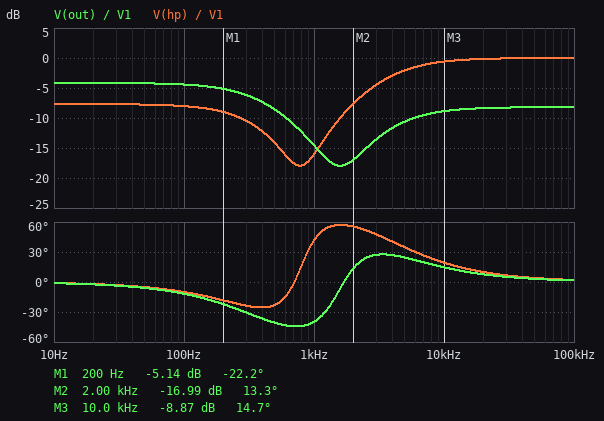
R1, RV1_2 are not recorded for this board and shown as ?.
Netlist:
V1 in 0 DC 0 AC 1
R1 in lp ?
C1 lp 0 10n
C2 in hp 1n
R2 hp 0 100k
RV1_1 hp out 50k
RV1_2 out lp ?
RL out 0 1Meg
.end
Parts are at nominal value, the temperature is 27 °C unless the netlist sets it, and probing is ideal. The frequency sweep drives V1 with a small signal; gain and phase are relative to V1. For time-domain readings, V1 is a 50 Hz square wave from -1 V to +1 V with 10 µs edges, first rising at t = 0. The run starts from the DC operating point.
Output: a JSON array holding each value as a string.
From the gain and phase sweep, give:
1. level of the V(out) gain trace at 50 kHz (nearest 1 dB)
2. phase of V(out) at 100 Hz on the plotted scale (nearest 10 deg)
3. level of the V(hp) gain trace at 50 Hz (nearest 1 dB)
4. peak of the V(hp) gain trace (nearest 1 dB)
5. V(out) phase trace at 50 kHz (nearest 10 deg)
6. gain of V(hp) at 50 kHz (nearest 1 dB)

["-8 dB", "-10 deg", "-8 dB", "0 dB", "0 deg", "0 dB"]
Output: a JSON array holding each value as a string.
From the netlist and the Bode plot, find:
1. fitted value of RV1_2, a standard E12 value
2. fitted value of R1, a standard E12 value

["33 kΩ", "47 kΩ"]
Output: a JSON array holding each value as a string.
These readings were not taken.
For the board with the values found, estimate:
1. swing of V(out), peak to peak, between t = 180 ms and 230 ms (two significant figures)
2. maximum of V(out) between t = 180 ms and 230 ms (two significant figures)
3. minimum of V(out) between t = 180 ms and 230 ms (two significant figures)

["1.2 V", "620 mV", "-620 mV"]
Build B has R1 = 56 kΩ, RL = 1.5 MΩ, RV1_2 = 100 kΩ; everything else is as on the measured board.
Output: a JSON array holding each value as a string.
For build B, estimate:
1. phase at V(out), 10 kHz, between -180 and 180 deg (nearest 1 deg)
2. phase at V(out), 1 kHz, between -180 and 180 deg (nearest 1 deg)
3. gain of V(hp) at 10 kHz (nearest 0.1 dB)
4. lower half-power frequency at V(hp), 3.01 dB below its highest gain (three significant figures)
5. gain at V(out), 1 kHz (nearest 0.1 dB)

["14 deg", "28 deg", "-0.3 dB", "2.93 kHz", "-17.0 dB"]
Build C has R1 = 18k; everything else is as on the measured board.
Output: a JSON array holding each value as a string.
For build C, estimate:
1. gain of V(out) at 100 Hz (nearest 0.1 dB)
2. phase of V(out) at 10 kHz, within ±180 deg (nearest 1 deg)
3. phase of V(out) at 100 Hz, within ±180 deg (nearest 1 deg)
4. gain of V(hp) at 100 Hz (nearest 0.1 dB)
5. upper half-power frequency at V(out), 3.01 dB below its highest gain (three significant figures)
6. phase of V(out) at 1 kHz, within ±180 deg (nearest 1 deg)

["-2.9 dB", "9 deg", "-5 deg", "-6.5 dB", "821 Hz", "-35 deg"]
